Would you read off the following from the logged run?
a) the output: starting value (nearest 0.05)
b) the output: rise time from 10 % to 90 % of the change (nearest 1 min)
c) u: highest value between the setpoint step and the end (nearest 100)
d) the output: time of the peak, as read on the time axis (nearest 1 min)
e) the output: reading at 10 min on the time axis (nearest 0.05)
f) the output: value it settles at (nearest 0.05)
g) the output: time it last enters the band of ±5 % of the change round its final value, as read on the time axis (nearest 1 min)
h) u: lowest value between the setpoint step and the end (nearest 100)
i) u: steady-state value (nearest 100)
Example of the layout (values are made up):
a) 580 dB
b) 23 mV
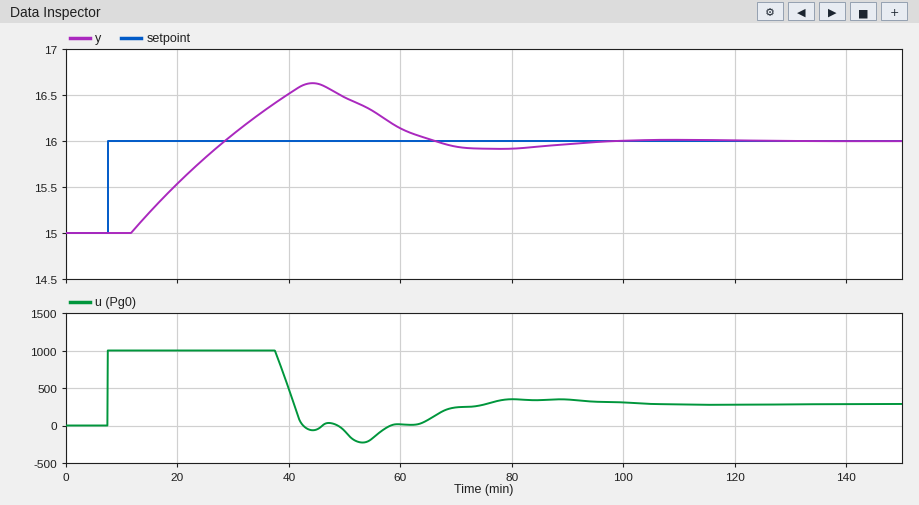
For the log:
a) 15.00
b) 13 min
c) 1000
d) 44 min
e) 15.00
f) 16.00
g) 87 min
h) -200
i) 300
